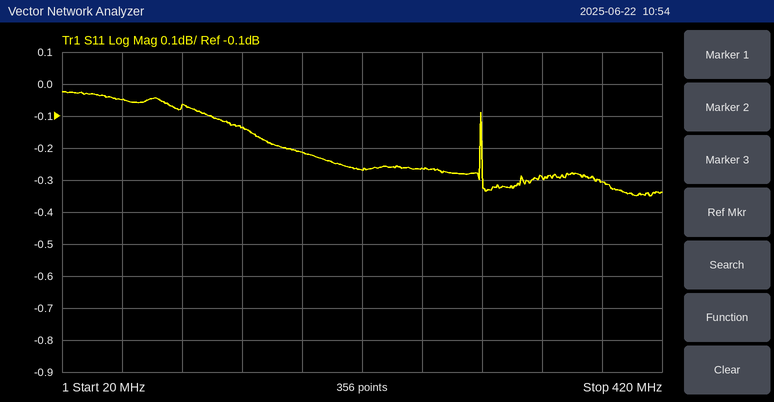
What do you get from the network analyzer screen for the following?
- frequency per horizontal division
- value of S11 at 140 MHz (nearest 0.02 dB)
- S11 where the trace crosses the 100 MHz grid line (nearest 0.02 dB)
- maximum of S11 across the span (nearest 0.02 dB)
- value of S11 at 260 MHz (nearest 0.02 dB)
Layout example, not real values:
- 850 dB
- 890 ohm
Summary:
- 40 MHz
- -0.14 dB
- -0.06 dB
- -0.02 dB
- -0.26 dB
